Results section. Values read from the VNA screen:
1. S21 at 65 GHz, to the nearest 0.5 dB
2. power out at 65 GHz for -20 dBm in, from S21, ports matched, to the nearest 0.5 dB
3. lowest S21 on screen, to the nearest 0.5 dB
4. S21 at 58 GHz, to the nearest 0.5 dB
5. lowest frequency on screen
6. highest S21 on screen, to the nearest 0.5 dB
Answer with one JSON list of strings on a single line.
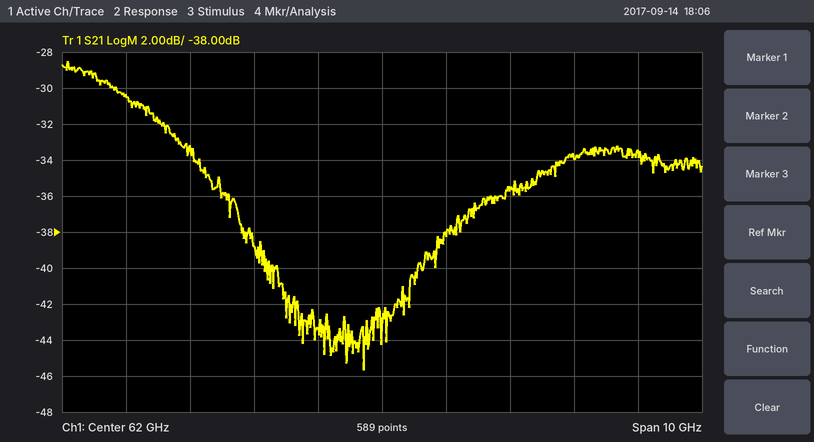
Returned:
["-34.0 dB", "-54.0 dBm", "-45.5 dB", "-30.5 dB", "57 GHz", "-28.5 dB"]
